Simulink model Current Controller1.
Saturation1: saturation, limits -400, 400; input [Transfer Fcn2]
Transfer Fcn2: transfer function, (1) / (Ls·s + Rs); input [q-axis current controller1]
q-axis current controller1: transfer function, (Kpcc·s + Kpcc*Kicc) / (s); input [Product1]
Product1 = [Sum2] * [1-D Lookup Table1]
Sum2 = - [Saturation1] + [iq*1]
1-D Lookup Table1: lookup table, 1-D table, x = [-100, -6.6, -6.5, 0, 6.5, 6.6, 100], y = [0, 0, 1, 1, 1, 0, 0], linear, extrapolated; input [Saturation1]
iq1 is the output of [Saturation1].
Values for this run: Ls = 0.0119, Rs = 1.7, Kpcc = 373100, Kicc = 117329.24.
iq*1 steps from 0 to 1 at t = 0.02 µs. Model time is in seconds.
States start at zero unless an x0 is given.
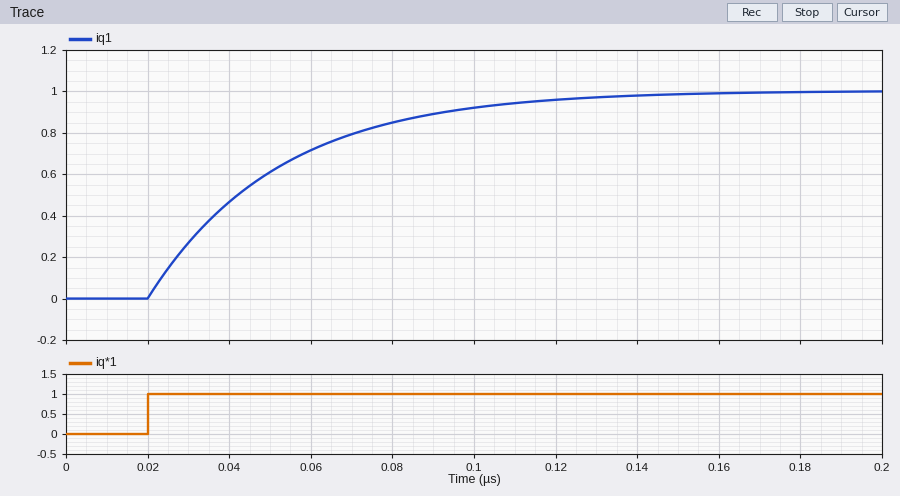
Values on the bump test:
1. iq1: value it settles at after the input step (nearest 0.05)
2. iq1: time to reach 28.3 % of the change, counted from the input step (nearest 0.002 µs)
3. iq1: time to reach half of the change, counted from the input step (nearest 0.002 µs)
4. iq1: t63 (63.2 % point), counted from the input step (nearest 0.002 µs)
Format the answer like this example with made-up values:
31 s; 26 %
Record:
1.00; 0.010 µs; 0.022 µs; 0.032 µs
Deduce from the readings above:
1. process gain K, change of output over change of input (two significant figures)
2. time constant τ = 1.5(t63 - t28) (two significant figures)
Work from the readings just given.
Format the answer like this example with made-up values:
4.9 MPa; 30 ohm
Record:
1.0; 0.033 µs
